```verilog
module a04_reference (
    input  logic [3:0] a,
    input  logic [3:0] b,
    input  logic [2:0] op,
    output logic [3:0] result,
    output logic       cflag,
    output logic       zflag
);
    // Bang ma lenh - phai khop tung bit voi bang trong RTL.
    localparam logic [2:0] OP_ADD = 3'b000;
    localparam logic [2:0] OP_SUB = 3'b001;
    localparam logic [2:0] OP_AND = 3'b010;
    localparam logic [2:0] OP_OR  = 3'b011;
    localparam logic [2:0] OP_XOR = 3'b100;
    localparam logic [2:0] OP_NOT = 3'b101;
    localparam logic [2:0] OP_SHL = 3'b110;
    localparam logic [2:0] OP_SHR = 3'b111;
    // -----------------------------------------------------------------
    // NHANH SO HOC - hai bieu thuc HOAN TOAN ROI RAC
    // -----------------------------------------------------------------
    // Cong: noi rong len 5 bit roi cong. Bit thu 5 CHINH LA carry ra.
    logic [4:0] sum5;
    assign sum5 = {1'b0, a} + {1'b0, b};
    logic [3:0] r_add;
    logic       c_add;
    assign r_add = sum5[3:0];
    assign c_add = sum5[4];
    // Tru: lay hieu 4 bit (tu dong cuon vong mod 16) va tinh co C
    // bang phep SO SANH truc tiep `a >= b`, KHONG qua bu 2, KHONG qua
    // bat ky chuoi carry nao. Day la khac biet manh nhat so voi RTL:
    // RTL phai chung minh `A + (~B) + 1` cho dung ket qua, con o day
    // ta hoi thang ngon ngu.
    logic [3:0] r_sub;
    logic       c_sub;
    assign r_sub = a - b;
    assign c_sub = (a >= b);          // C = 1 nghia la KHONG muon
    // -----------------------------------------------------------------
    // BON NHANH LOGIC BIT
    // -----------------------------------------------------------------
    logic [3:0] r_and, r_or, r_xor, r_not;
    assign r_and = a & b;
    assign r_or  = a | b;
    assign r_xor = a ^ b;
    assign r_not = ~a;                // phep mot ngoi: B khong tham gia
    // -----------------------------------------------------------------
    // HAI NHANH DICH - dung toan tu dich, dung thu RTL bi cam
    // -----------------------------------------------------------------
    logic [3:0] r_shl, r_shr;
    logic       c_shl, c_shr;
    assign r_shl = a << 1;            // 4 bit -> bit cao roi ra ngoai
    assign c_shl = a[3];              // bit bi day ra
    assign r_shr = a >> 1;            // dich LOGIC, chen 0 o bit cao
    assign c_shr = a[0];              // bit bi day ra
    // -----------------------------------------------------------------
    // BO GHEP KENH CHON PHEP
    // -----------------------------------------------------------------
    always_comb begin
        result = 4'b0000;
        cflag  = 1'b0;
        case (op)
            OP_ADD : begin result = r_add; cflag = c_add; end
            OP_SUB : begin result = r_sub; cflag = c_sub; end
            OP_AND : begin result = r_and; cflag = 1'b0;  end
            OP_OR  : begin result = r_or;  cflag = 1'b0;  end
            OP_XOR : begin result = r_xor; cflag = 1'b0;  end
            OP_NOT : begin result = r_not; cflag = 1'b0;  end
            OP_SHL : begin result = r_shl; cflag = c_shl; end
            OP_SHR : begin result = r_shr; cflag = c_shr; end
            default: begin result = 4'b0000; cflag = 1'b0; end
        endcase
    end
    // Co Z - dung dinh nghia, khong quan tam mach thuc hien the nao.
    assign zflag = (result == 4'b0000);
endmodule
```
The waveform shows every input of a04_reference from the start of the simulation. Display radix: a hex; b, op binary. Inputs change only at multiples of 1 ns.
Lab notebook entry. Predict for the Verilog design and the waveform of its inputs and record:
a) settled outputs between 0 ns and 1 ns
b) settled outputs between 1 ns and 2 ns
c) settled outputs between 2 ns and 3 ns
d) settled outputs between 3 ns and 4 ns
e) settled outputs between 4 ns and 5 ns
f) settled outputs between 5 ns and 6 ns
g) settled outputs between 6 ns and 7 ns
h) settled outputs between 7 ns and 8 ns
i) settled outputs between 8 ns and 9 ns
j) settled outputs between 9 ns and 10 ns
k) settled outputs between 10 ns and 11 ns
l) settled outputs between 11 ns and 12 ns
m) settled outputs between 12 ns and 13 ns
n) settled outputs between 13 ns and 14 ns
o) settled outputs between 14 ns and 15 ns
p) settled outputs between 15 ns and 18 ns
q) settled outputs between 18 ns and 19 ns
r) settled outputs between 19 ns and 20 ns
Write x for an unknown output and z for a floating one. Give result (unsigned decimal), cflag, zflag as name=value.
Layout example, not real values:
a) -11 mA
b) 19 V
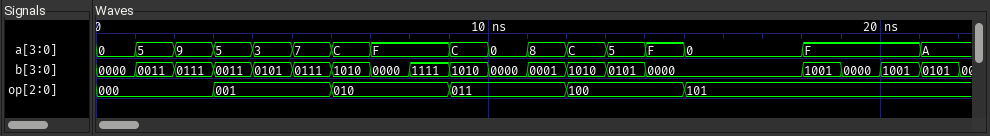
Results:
a) result=0, cflag=0, zflag=1
b) result=8, cflag=0, zflag=0
c) result=0, cflag=1, zflag=1
d) result=2, cflag=1, zflag=0
e) result=14, cflag=0, zflag=0
f) result=0, cflag=1, zflag=1
g) result=8, cflag=0, zflag=0
h) result=0, cflag=0, zflag=1
i) result=15, cflag=0, zflag=0
j) result=14, cflag=0, zflag=0
k) result=0, cflag=0, zflag=1
l) result=9, cflag=0, zflag=0
m) result=6, cflag=0, zflag=0
n) result=0, cflag=0, zflag=1
o) result=15, cflag=0, zflag=0
p) result=15, cflag=0, zflag=0
q) result=0, cflag=0, zflag=1
r) result=0, cflag=0, zflag=1
